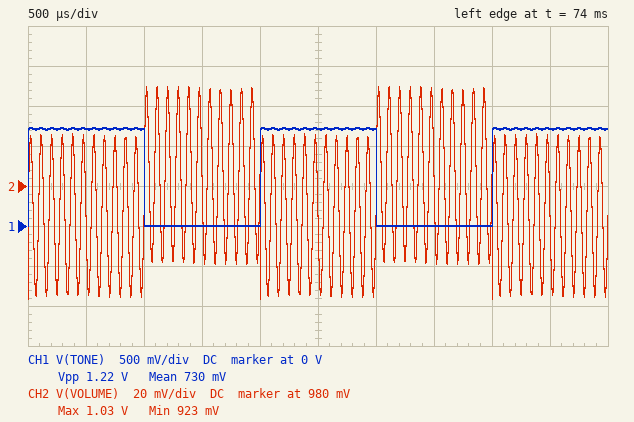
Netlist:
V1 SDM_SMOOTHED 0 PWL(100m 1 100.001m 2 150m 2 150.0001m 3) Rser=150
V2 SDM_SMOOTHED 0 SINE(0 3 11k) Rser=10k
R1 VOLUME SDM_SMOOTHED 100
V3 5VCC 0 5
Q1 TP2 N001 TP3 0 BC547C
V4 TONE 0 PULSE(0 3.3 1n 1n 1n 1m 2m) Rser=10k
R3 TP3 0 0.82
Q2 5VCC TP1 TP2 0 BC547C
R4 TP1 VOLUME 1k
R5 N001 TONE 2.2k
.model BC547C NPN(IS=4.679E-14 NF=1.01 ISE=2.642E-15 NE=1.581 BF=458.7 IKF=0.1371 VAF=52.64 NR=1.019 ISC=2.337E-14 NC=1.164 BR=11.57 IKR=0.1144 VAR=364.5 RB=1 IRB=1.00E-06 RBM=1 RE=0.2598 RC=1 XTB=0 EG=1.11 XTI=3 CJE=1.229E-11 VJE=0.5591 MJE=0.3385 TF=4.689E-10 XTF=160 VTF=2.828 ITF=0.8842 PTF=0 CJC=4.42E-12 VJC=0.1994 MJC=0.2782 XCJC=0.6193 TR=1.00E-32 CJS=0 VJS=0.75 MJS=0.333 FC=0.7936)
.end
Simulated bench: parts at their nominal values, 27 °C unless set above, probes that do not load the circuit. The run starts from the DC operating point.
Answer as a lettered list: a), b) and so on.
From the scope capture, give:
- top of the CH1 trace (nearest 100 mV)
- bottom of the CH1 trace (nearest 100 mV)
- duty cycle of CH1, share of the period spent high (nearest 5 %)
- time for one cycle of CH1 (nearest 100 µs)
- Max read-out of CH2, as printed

a) 1.2 V
b) 0 V
c) 50 %
d) 2.0 ms
e) 1.03 V
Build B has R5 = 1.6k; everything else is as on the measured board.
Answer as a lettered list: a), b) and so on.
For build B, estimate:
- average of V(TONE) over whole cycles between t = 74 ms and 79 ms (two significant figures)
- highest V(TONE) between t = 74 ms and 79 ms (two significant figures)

a) 550 mV
b) 1.1 V
